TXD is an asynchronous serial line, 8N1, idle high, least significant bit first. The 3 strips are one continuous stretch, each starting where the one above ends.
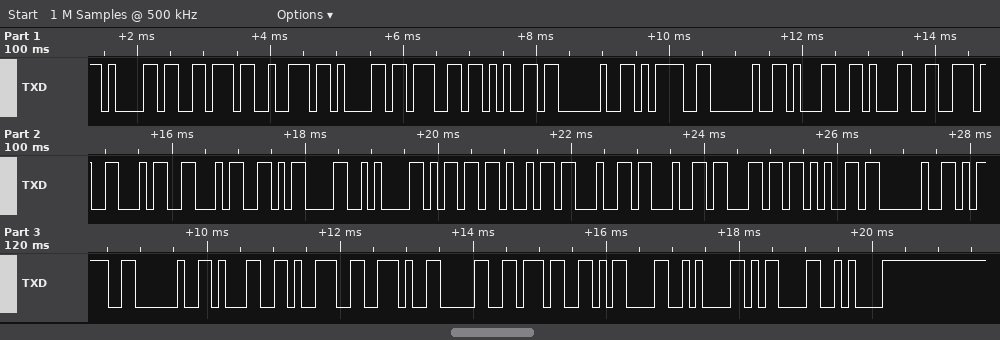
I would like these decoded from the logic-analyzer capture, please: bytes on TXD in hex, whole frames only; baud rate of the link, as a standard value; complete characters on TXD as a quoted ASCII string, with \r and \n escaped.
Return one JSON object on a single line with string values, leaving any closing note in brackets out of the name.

{"bytes on TXD in hex, whole frames only": "61 76 72 61 67 65 20 3D 20 31 31 2E 34 34 0D 0A 6D 69 64 64 6C 65 20 3D 20 31 39 2E 30 37 0D 0A 0D 0A", "baud rate of the link, as a standard value": "9600 baud", "complete characters on TXD as a quoted ASCII string, with \\r and \\n escaped": "\"avrage = 11.44\\r\\nmiddle = 19.07\\r\\n\\r\\n\""}
